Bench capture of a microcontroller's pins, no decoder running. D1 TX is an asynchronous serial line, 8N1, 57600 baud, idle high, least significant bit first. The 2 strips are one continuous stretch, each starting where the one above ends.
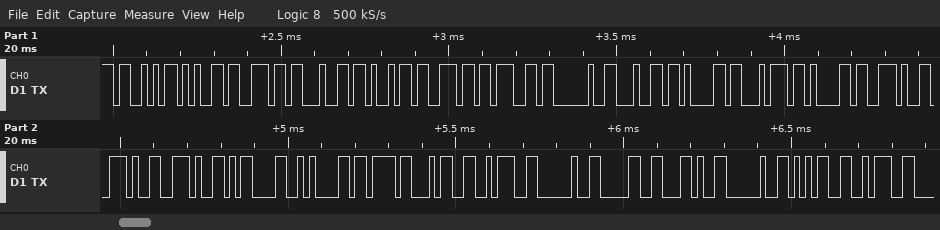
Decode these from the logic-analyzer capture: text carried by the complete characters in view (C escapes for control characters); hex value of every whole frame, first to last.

"Sending data...\r\n{4: 0, 5:"
53 65 6E 64 69 6E 67 20 64 61 74 61 2E 2E 2E 0D 0A 7B 34 3A 20 30 2C 20 35 3A
